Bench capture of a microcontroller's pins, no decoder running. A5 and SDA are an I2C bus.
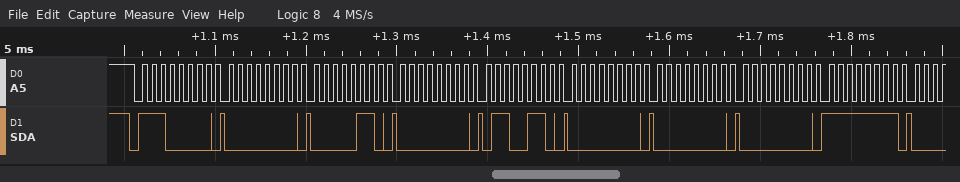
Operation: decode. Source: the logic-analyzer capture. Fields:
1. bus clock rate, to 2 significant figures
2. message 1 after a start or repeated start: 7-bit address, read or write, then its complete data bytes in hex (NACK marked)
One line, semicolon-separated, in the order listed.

100 kHz; 0x70 write: 00 06 00 66 00 00 00 FF
